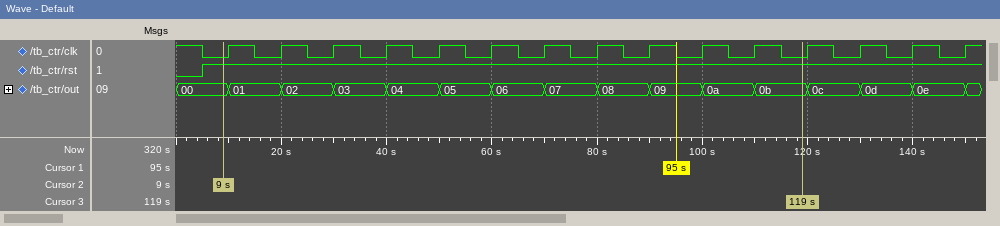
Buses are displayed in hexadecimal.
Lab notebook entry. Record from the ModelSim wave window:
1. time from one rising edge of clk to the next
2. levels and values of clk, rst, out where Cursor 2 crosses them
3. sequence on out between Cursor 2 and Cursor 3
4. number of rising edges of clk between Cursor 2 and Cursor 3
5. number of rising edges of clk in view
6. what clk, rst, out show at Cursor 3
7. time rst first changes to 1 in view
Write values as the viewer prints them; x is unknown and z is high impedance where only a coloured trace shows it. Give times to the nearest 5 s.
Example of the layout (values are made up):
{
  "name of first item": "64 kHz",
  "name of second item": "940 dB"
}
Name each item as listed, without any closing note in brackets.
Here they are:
{
  "time from one rising edge of clk to the next": "10 s",
  "levels and values of clk, rst, out where Cursor 2 crosses them": "clk=0, rst=1, out=00",
  "sequence on out between Cursor 2 and Cursor 3": "00, 01, 02, 03, 04, 05, 06, 07, 08, 09, 0a, 0b",
  "number of rising edges of clk between Cursor 2 and Cursor 3": "11",
  "number of rising edges of clk in view": "15",
  "what clk, rst, out show at Cursor 3": "clk=0, rst=1, out=0b",
  "time rst first changes to 1 in view": "5 s"
}
